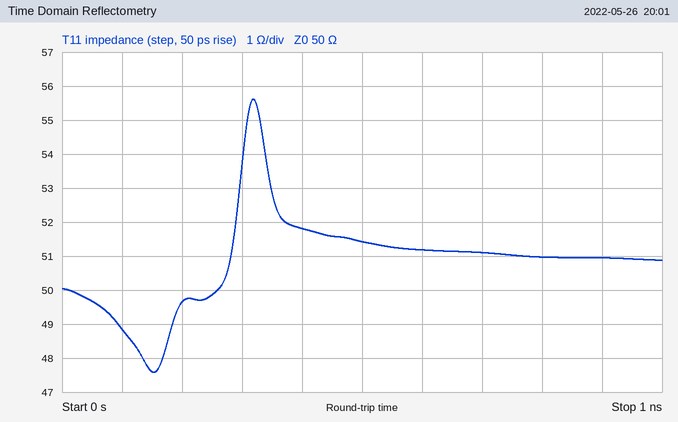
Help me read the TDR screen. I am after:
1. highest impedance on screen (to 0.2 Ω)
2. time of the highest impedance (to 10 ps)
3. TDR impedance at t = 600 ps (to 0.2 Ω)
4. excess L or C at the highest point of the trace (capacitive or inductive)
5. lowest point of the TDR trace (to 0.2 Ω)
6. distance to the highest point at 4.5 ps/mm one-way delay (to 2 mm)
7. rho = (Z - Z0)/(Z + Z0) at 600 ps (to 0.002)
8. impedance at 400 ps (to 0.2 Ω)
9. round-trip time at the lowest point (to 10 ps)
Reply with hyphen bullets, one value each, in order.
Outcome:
- 55.6 Ω
- 320 ps
- 51.2 Ω
- inductive
- 47.6 Ω
- 36 mm
- +0.012
- 51.8 Ω
- 150 ps
